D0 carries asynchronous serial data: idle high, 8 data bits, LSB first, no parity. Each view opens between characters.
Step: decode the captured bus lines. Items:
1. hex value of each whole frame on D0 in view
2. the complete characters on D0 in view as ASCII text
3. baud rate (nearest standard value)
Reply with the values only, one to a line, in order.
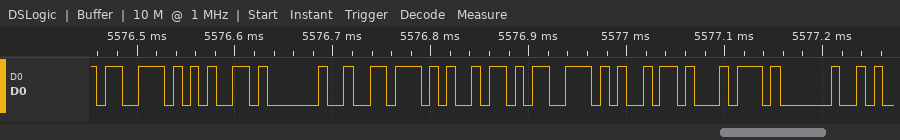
73, 65, 20, 76, 69, 73, 69, 74, 20
"se visit "
115200 baud
